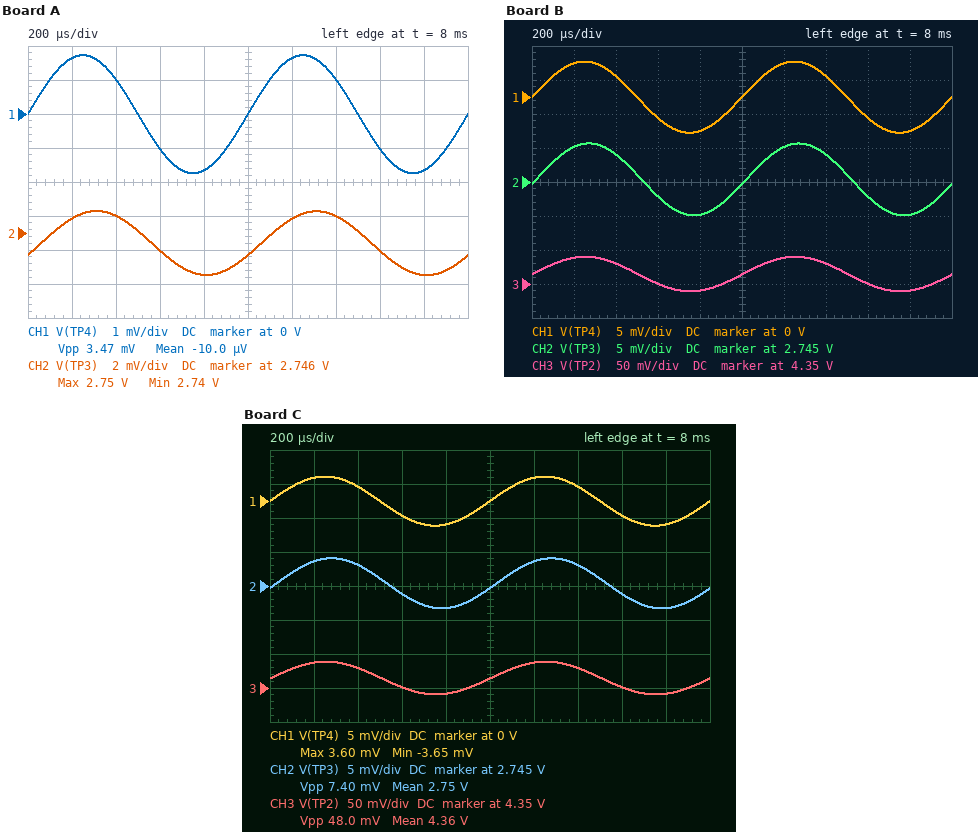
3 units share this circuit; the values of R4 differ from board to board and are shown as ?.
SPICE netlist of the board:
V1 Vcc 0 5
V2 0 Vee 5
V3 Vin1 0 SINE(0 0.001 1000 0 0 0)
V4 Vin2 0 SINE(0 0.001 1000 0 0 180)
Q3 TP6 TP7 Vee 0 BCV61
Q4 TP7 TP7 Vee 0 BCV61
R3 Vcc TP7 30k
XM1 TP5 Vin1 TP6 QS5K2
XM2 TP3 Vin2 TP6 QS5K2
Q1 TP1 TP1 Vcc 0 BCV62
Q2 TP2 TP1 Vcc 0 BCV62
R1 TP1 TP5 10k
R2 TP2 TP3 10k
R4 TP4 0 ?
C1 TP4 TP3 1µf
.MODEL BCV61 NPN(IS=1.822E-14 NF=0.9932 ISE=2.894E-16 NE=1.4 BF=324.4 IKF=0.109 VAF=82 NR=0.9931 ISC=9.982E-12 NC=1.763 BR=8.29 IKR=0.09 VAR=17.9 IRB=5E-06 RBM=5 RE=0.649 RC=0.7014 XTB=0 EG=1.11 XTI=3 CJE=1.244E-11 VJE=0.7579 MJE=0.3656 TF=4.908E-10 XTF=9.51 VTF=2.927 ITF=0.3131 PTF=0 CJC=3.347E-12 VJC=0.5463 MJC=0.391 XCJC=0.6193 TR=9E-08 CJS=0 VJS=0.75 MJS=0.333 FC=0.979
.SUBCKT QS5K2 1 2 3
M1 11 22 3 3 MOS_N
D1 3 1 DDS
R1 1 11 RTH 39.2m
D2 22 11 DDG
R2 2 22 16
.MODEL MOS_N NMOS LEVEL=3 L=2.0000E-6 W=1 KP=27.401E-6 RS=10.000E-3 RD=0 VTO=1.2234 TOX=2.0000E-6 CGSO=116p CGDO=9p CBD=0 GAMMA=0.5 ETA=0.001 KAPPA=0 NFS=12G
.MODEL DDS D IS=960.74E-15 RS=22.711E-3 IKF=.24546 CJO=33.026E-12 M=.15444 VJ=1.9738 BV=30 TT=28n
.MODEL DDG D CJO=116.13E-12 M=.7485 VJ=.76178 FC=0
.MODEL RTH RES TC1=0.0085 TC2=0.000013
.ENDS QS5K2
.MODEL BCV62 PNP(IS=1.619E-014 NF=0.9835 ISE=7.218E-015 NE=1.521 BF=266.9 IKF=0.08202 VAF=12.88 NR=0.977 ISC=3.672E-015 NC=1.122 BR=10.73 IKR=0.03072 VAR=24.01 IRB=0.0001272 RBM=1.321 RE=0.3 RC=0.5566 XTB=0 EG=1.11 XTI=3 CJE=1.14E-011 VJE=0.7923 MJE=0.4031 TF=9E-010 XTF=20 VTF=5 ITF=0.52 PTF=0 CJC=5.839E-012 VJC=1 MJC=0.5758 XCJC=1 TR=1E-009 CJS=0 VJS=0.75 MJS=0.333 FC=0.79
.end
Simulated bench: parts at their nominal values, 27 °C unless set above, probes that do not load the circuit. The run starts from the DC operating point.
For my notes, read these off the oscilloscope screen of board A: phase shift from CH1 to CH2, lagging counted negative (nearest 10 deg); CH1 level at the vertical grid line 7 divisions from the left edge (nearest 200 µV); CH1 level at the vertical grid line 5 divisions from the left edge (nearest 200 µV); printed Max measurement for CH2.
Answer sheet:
-20 deg
1.0 mV
0 V
2.75 V
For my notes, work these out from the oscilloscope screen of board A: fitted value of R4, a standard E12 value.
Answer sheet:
390 Ω
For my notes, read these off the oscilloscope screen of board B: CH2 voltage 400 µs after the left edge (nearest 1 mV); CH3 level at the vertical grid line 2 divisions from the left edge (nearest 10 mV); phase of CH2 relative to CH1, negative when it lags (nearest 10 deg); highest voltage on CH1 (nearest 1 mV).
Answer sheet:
2.749 V
4.38 V
-10 deg
5 mV
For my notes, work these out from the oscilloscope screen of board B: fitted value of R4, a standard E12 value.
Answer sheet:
1.2 kΩ
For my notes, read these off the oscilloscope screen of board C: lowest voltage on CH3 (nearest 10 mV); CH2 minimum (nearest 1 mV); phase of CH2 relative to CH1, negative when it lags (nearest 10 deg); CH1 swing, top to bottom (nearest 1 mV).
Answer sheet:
4.34 V
2.742 V
-10 deg
7 mV
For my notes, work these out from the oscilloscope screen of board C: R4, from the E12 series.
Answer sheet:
820 Ω
